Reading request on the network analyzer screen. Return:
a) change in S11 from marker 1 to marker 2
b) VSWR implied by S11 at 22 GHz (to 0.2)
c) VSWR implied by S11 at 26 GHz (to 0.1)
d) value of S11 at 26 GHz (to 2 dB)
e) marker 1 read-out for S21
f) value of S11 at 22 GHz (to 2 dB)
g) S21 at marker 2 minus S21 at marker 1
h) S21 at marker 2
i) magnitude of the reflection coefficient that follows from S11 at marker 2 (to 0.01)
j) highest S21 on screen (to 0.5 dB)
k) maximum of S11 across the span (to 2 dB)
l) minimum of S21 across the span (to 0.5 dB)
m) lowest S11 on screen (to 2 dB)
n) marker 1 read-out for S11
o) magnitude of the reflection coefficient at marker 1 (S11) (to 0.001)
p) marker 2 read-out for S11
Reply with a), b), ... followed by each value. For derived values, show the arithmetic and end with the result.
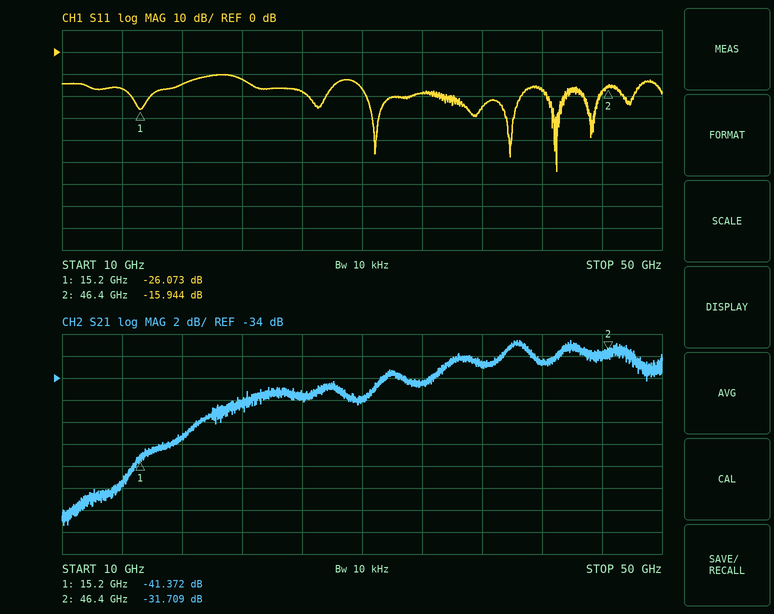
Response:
a) -15.944 − (-26.073) = 10.129 dB
b) |Γ| = 10^(-12/20) = 0.2512; VSWR = (1 + 0.2512)/(1 − 0.2512) ≈ 1.67, so 1.6 to the nearest 0.2
c) |Γ| = 10^(-18/20) = 0.1259; VSWR = (1 + 0.1259)/(1 − 0.1259) ≈ 1.3
d) -18 dB
e) -41.372 dB
f) -12 dB
g) -31.709 − (-41.372) = 9.663 dB
h) -31.709 dB
i) 10^(-15.944/20) ≈ 0.16
j) -30.5 dB
k) -10 dB
l) -47.5 dB
m) -54 dB
n) -26.073 dB
o) 10^(-26.073/20) ≈ 0.050
p) -15.944 dB
